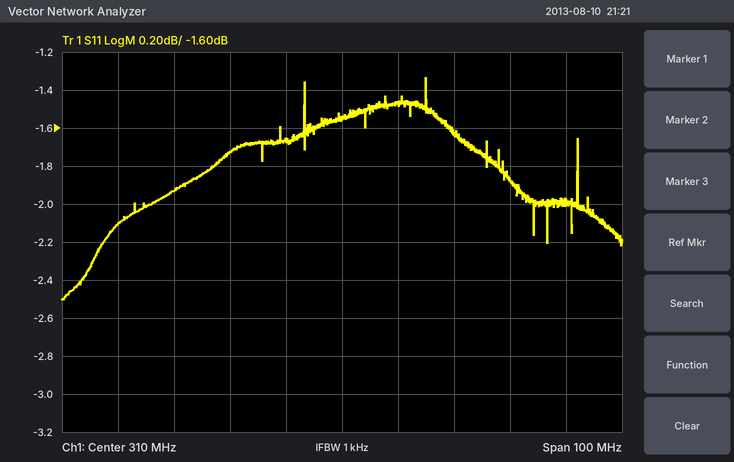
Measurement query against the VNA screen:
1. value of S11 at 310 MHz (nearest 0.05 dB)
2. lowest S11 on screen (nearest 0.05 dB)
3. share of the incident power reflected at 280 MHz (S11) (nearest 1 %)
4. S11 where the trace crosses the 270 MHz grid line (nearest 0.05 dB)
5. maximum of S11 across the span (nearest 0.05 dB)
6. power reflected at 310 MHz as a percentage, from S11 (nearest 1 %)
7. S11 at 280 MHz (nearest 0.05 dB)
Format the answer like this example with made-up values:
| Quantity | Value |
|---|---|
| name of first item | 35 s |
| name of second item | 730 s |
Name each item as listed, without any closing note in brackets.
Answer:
| Quantity | Value |
|---|---|
| value of S11 at 310 MHz | -1.55 dB |
| lowest S11 on screen | -2.50 dB |
| share of the incident power reflected at 280 MHz (S11) | 64 % |
| S11 where the trace crosses the 270 MHz grid line | -2.10 dB |
| maximum of S11 across the span | -1.35 dB |
| power reflected at 310 MHz as a percentage, from S11 | 70 % |
| S11 at 280 MHz | -1.95 dB |
